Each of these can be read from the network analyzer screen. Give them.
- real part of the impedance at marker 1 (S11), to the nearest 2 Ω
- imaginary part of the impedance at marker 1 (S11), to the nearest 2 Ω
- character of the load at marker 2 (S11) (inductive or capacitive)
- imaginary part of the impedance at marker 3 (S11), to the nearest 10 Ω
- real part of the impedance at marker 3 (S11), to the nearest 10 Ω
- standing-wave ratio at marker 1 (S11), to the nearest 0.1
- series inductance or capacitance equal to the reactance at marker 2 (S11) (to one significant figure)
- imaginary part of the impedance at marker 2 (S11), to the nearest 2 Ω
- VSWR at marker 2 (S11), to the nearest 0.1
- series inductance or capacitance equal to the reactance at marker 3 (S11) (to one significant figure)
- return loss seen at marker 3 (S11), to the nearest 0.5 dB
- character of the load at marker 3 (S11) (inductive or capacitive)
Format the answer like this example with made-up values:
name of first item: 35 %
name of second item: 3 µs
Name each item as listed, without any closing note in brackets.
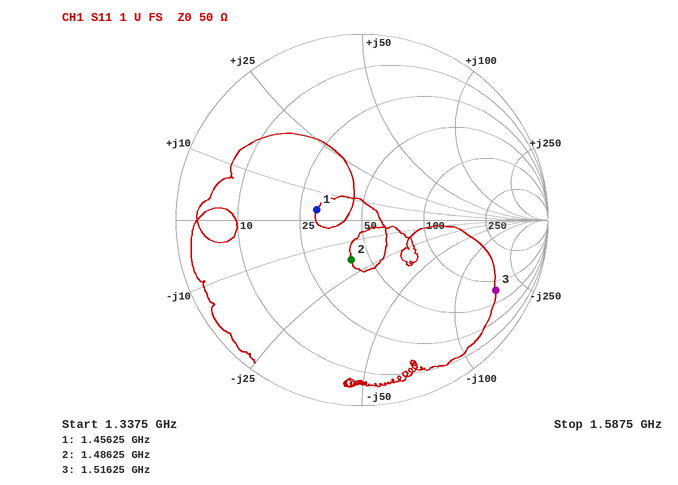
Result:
real part of the impedance at marker 1 (S11), to the nearest 2 Ω: 30 Ω
imaginary part of the impedance at marker 1 (S11), to the nearest 2 Ω: +4 Ω
character of the load at marker 2 (S11): capacitive
imaginary part of the impedance at marker 3 (S11), to the nearest 10 Ω: -170 Ω
real part of the impedance at marker 3 (S11), to the nearest 10 Ω: 80 Ω
standing-wave ratio at marker 1 (S11), to the nearest 0.1: 1.7
series inductance or capacitance equal to the reactance at marker 2 (S11): 6 pF
imaginary part of the impedance at marker 2 (S11), to the nearest 2 Ω: -18 Ω
VSWR at marker 2 (S11), to the nearest 0.1: 1.6
series inductance or capacitance equal to the reactance at marker 3 (S11): 600 fF
return loss seen at marker 3 (S11), to the nearest 0.5 dB: 2.0 dB
character of the load at marker 3 (S11): capacitive
